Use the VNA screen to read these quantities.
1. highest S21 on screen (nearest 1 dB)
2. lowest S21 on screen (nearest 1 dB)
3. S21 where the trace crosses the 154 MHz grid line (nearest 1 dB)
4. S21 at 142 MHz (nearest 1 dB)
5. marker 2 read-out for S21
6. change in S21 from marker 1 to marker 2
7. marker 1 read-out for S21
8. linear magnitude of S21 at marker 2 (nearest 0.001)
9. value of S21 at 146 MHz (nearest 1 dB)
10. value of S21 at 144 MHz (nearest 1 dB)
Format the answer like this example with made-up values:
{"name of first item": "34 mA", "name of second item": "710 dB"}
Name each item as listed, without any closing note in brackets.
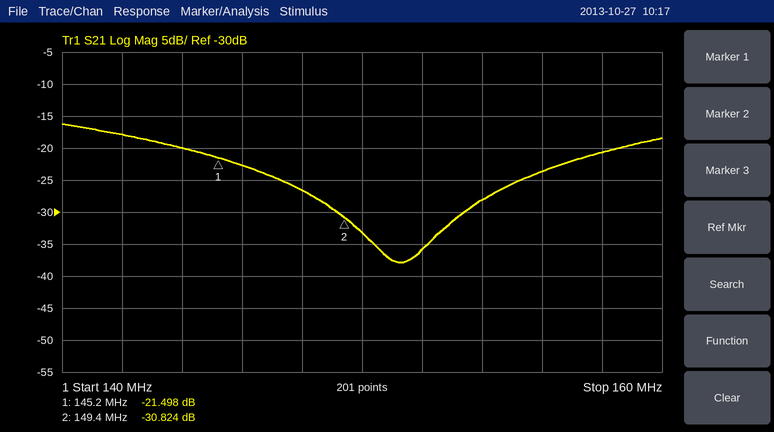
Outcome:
{"highest S21 on screen": "-16 dB", "lowest S21 on screen": "-38 dB", "S21 where the trace crosses the 154 MHz grid line": "-28 dB", "S21 at 142 MHz": "-18 dB", "marker 2 read-out for S21": "-30.824 dB", "change in S21 from marker 1 to marker 2": "-9.326 dB", "marker 1 read-out for S21": "-21.498 dB", "linear magnitude of S21 at marker 2": "0.029", "value of S21 at 146 MHz": "-23 dB", "value of S21 at 144 MHz": "-20 dB"}
